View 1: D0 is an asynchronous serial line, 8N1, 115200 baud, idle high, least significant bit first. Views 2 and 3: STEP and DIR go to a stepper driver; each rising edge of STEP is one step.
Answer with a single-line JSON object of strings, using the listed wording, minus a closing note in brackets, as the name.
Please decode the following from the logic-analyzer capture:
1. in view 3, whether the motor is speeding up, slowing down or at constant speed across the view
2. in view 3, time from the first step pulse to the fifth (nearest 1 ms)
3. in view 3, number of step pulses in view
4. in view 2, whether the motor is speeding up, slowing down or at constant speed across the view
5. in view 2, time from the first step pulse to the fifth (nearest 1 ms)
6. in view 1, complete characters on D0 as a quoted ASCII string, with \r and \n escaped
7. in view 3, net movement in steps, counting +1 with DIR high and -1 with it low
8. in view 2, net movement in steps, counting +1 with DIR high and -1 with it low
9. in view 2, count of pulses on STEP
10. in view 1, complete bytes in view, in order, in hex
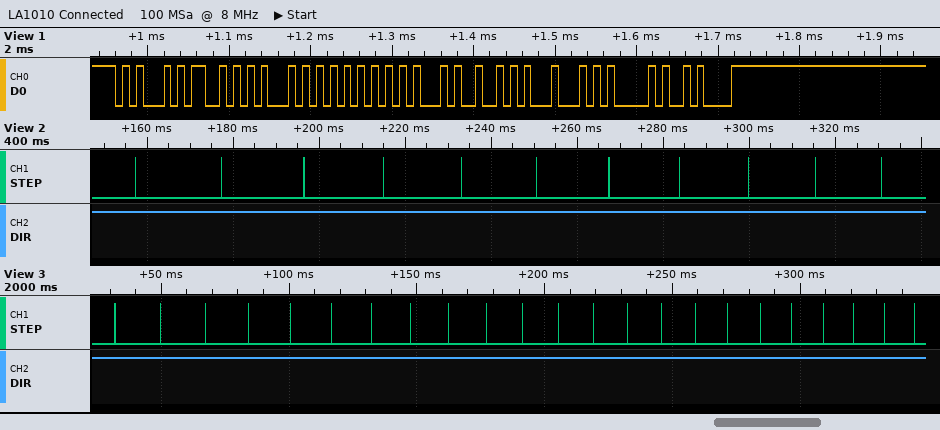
{"in view 3, whether the motor is speeding up, slowing down or at constant speed across the view": "speeding up", "in view 3, time from the first step pulse to the fifth": "69 ms", "in view 3, number of step pulses in view": "23", "in view 2, whether the motor is speeding up, slowing down or at constant speed across the view": "speeding up", "in view 2, time from the first step pulse to the fifth": "76 ms", "in view 1, complete characters on D0 as a quoted ASCII string, with \\r and \\n escaped": "\"ESQUERDA\\n\"", "in view 3, net movement in steps, counting +1 with DIR high and -1 with it low": "+23", "in view 2, net movement in steps, counting +1 with DIR high and -1 with it low": "+11", "in view 2, count of pulses on STEP": "11", "in view 1, complete bytes in view, in order, in hex": "0x45 0x53 0x51 0x55 0x45 0x52 0x44 0x41 0x0A"}
